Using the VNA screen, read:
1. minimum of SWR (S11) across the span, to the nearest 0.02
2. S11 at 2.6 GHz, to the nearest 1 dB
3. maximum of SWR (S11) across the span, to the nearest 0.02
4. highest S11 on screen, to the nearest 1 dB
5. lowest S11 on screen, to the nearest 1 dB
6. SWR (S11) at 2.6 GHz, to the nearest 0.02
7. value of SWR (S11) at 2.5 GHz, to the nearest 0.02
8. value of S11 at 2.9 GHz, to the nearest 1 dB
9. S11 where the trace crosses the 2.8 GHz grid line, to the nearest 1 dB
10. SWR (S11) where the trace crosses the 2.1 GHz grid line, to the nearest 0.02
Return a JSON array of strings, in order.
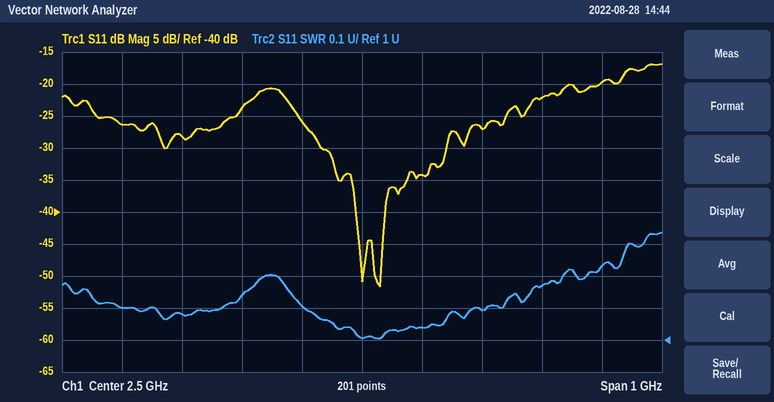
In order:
["1.00", "-34 dB", "1.34", "-17 dB", "-52 dB", "1.04", "1.00", "-20 dB", "-22 dB", "1.10"]
